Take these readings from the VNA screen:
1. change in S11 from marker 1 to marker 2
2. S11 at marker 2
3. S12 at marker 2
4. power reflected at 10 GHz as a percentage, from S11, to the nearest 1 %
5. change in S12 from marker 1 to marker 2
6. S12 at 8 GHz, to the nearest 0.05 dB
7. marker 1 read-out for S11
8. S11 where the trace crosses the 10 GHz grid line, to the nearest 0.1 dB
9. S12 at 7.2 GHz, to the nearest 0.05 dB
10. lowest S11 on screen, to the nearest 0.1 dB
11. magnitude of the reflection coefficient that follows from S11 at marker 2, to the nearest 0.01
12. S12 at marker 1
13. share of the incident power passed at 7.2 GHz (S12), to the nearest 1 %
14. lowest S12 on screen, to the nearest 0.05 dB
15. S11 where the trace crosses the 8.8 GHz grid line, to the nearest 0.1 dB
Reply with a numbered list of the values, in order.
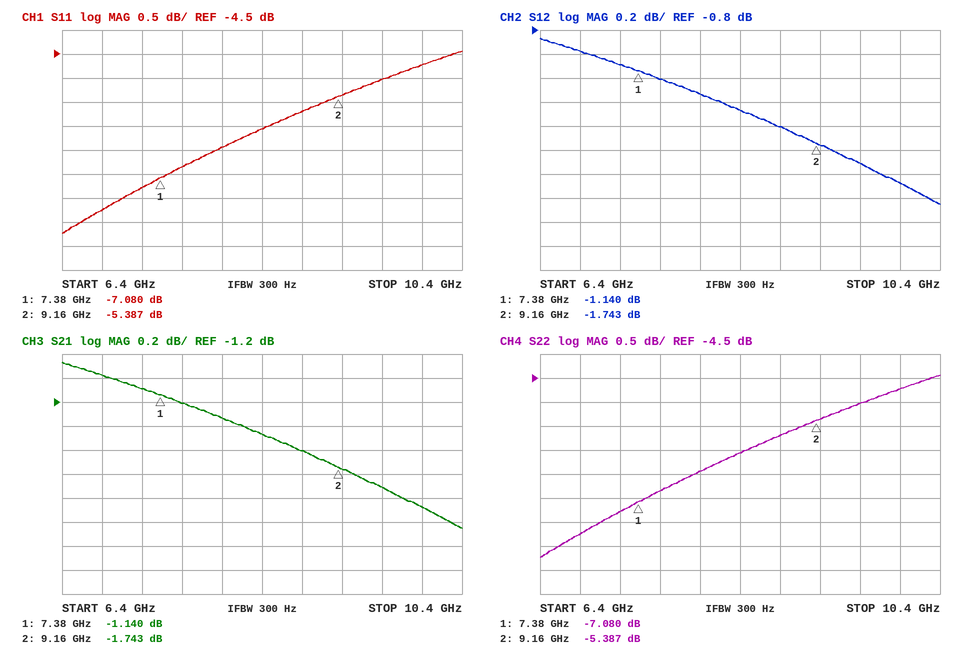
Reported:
1. 1.693 dB
2. -5.387 dB
3. -1.743 dB
4. 34 %
5. -0.603 dB
6. -1.35 dB
7. -7.080 dB
8. -4.7 dB
9. -1.10 dB
10. -8.2 dB
11. 0.54
12. -1.140 dB
13. 78 %
14. -2.25 dB
15. -5.7 dB
